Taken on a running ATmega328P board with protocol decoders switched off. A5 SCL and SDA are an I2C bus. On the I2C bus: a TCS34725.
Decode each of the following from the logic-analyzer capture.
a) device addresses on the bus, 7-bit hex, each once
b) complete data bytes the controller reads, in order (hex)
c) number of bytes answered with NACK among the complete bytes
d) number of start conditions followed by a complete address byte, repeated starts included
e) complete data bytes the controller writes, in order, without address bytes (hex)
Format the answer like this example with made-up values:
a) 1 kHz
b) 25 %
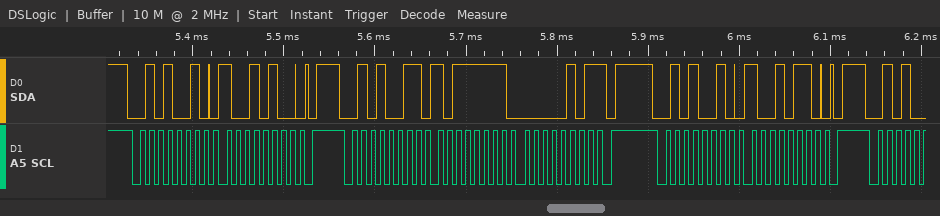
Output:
a) 0x29
b) BF 05
c) 1
d) 3
e) 94 96
